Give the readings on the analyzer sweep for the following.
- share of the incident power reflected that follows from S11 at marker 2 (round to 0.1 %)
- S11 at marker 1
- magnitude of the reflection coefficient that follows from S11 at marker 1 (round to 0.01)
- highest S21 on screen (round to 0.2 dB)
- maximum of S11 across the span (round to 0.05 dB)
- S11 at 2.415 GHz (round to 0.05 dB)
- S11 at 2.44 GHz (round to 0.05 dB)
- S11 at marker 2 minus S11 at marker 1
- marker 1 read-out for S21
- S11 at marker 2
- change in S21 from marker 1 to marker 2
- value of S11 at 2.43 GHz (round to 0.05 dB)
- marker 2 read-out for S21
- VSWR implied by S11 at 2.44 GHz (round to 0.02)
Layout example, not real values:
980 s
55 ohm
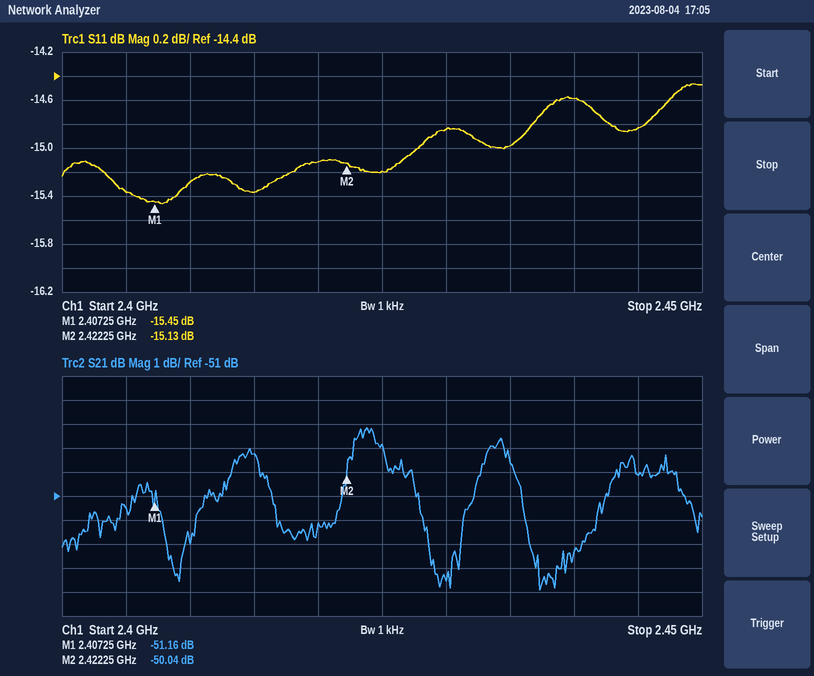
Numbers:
3.1 %
-15.45 dB
0.17
-48.2 dB
-14.45 dB
-15.35 dB
-14.60 dB
0.32 dB
-51.16 dB
-15.13 dB
1.12 dB
-14.85 dB
-50.04 dB
1.46
